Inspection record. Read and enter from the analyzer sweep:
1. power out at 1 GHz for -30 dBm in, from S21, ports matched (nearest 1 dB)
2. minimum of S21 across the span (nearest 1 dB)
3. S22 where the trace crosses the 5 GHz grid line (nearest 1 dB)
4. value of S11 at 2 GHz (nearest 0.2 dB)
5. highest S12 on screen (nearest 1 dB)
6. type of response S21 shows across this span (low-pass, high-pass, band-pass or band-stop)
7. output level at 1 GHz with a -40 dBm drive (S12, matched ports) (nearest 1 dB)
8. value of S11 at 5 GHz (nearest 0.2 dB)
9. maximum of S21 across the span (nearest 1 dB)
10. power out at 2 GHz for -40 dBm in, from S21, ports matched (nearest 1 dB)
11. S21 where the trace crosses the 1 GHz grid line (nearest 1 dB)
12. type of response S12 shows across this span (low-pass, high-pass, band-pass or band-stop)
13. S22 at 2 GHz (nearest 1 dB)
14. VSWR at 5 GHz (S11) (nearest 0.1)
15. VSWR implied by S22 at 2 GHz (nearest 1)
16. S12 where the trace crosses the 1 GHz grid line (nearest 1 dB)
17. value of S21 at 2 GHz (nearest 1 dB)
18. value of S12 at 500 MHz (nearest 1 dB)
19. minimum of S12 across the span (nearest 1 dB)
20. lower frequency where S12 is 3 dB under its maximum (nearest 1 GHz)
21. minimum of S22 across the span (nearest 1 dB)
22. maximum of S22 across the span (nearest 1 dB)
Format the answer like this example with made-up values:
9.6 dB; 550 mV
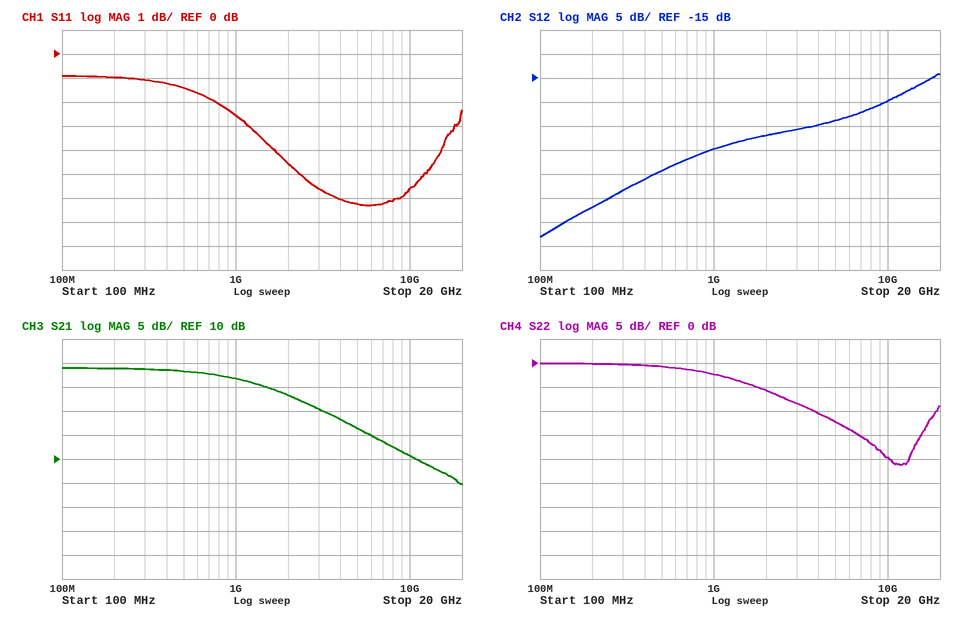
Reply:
-3 dBm; 5 dB; -12 dB; -4.6 dB; -14 dB; low-pass; -70 dBm; -6.2 dB; 29 dB; -17 dBm; 27 dB; high-pass; -6 dB; 2.9; 3; -30 dB; 23 dB; -34 dB; -48 dB; 14 GHz; -21 dB; 0 dB
